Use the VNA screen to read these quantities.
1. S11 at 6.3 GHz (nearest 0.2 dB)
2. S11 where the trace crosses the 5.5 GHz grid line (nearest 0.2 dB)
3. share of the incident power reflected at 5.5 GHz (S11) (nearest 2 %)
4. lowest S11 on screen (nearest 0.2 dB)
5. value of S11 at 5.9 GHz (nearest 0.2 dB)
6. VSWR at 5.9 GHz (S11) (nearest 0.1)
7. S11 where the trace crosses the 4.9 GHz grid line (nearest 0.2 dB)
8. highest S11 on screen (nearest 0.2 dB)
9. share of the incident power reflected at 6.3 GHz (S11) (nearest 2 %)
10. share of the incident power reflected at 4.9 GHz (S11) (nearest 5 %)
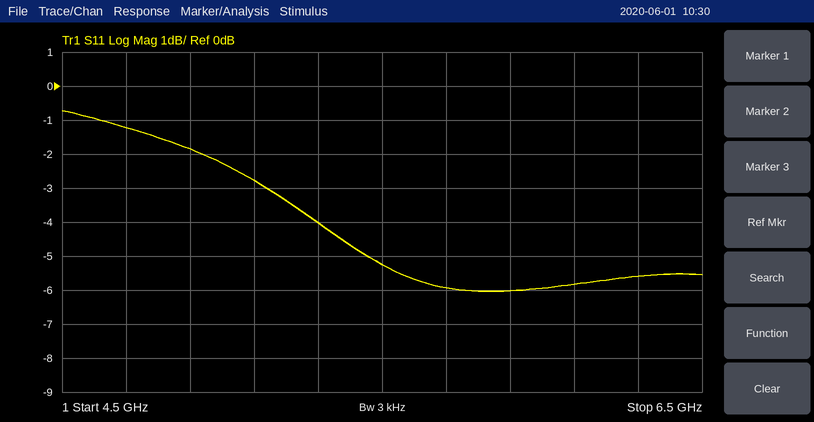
-5.6 dB
-5.2 dB
30 %
-6.0 dB
-6.0 dB
3.0
-1.8 dB
-0.8 dB
28 %
65 %
